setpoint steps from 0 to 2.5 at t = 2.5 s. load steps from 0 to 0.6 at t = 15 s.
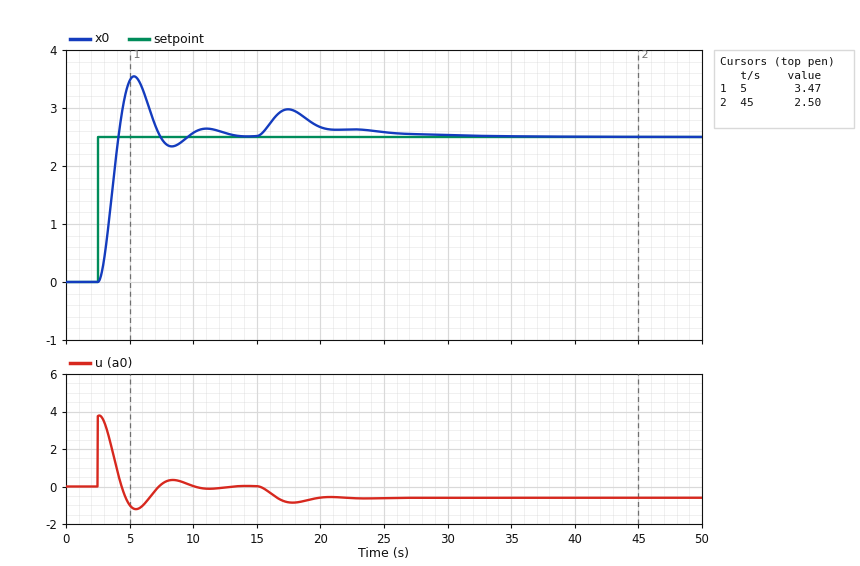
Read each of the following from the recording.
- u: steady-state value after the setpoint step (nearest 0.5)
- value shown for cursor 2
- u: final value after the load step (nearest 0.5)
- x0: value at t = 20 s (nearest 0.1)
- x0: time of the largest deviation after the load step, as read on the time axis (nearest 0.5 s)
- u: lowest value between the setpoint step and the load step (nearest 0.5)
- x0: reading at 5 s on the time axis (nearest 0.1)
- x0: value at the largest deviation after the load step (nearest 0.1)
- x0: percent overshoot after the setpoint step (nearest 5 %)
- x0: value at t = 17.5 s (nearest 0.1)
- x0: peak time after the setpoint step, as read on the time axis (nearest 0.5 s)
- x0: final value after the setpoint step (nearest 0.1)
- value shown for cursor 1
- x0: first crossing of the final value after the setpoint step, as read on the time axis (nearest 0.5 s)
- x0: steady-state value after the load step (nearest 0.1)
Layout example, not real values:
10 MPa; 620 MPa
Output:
0.0; 2.50; -0.5; 2.7; 17.5 s; -1.0; 3.5; 3.0; 40 %; 3.0; 5.5 s; 2.5; 3.47; 4.0 s; 2.5
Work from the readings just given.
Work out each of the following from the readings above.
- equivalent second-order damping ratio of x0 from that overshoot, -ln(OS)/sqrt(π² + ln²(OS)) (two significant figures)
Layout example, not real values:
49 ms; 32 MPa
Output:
0.28
